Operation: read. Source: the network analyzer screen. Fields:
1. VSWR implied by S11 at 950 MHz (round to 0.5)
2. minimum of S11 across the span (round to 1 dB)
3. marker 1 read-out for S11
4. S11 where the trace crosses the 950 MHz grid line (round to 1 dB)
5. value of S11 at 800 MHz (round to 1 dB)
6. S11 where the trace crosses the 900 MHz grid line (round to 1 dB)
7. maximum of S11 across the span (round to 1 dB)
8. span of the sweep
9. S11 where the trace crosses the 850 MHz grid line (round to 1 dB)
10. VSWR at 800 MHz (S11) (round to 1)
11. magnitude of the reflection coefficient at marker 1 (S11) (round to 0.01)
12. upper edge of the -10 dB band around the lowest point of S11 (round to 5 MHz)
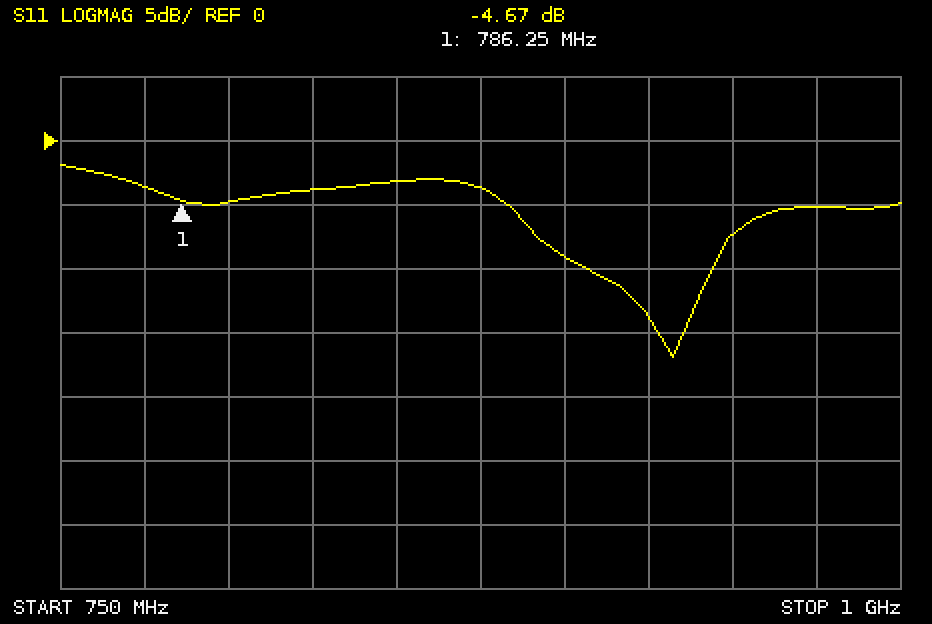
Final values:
2.5
-17 dB
-4.67 dB
-7 dB
-5 dB
-9 dB
-2 dB
250 MHz
-3 dB
4
0.58
945 MHz
